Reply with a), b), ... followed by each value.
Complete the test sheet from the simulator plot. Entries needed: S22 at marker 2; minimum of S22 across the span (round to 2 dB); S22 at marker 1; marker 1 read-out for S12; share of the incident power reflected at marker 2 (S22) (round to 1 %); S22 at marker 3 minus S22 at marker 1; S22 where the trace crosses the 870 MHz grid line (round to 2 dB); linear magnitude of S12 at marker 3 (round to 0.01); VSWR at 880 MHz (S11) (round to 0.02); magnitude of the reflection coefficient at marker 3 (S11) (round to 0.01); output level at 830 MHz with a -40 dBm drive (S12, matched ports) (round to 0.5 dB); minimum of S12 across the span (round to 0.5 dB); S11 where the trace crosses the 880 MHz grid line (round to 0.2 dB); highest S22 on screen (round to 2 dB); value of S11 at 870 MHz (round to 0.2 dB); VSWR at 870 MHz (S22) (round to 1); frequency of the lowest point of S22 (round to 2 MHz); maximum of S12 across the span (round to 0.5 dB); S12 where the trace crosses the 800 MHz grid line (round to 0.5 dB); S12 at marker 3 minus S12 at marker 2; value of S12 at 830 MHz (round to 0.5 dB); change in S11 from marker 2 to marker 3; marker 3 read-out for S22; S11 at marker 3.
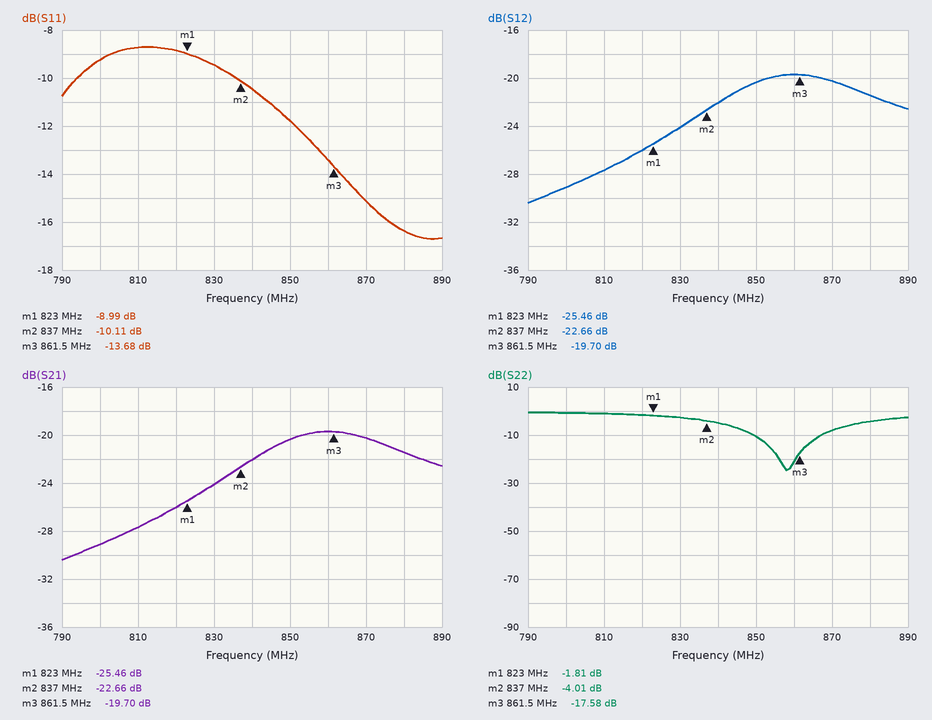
a) -4.01 dB
b) -24 dB
c) -1.81 dB
d) -25.46 dB
e) 40 %
f) -15.77 dB
g) -8 dB
h) 0.10
i) 1.36
j) 0.21
k) -64.0 dBm
l) -30.5 dB
m) -16.4 dB
n) 0 dB
o) -15.2 dB
p) 2
q) 858 MHz
r) -19.5 dB
s) -29.0 dB
t) 2.96 dB
u) -24.0 dB
v) -3.57 dB
w) -17.58 dB
x) -13.68 dB
